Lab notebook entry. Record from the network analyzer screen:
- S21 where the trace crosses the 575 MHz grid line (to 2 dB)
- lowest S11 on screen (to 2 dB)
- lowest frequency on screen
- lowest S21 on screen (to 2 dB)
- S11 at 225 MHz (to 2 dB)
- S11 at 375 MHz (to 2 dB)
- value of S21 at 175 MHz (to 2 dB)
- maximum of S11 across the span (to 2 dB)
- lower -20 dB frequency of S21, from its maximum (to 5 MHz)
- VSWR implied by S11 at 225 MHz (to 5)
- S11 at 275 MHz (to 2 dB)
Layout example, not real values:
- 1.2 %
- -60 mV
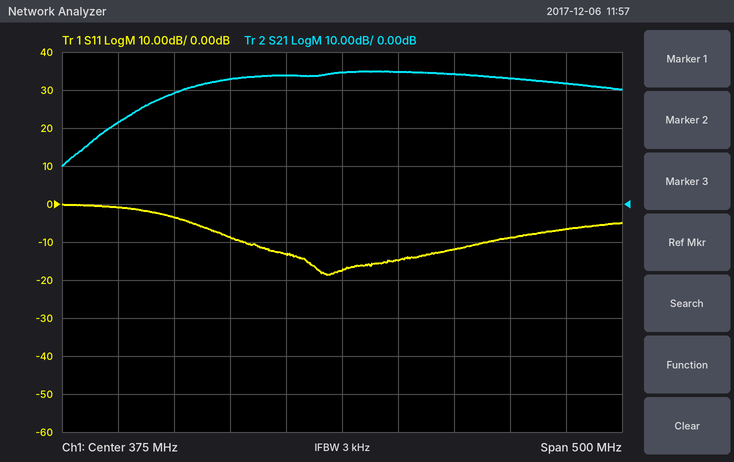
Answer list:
- 32 dB
- -18 dB
- 125 MHz
- 10 dB
- -4 dB
- -18 dB
- 22 dB
- 0 dB
- 145 MHz
- 5
- -8 dB
